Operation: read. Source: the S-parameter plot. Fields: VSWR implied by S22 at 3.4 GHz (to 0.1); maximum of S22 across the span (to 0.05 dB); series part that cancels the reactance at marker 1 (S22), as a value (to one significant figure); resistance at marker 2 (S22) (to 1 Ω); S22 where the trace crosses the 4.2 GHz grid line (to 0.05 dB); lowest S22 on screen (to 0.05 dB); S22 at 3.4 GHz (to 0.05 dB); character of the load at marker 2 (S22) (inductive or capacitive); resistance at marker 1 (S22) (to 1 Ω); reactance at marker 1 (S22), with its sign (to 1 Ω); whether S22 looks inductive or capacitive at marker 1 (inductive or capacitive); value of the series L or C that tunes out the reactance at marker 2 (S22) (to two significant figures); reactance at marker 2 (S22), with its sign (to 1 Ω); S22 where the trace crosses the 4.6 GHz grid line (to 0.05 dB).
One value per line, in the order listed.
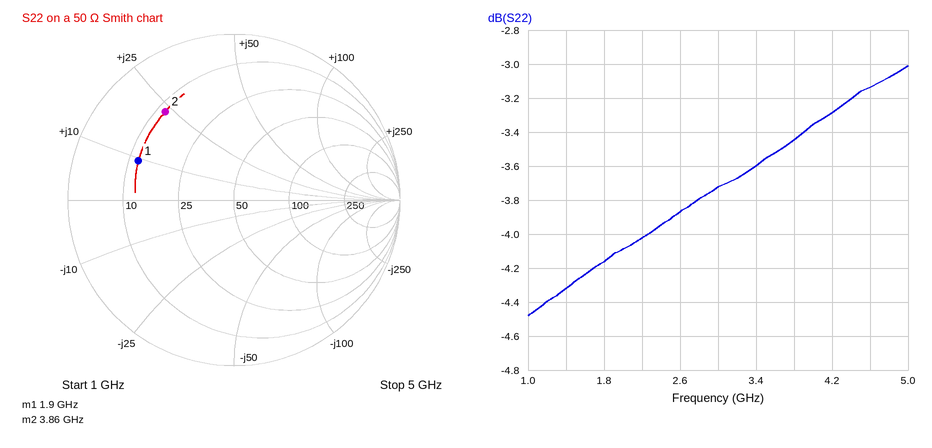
4.9
-3.00 dB
9 pF
12 Ω
-3.30 dB
-4.50 dB
-3.60 dB
inductive
12 Ω
+9 Ω
inductive
1.8 pF
+23 Ω
-3.15 dB
